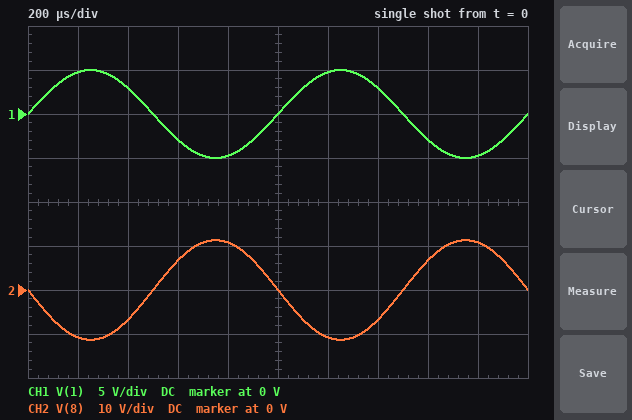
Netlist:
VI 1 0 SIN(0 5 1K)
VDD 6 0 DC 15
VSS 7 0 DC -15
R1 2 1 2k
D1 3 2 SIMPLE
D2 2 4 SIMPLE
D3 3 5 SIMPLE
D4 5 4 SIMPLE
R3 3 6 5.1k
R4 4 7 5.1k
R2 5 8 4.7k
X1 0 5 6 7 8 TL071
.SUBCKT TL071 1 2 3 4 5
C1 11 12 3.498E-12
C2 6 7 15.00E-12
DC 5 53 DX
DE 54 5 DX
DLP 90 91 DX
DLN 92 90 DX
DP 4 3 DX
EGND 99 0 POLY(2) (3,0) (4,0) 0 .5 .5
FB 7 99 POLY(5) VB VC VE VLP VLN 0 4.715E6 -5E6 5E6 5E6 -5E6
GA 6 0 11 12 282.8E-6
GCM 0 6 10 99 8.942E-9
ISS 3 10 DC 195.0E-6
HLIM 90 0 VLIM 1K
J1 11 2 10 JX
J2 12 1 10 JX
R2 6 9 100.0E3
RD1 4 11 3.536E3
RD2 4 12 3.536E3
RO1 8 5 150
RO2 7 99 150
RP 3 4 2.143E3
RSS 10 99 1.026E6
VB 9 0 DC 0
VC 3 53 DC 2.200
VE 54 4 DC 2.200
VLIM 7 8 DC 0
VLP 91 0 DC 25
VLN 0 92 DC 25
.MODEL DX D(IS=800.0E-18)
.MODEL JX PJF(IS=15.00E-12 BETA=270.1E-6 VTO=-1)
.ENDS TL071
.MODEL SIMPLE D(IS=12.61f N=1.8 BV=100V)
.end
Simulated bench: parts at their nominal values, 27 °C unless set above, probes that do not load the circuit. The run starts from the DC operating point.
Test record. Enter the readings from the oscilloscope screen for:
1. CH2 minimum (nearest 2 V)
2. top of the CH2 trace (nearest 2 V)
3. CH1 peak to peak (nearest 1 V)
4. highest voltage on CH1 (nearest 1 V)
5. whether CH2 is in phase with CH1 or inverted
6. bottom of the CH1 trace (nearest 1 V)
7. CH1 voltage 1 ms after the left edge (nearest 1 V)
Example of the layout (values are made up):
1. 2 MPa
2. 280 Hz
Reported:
1. -12 V
2. 12 V
3. 10 V
4. 5 V
5. inverted
6. -5 V
7. 0 V
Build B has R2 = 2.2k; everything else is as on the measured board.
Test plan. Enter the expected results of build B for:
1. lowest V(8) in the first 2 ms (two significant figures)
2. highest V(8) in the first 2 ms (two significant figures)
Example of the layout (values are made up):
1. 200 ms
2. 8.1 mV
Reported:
1. -5.3 V
2. 5.3 V
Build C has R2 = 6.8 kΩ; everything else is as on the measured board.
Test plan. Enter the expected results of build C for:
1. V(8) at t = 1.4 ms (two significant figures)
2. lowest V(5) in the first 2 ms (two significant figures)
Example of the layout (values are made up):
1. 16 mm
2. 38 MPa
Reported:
1. -9.8 V
2. -430 mV
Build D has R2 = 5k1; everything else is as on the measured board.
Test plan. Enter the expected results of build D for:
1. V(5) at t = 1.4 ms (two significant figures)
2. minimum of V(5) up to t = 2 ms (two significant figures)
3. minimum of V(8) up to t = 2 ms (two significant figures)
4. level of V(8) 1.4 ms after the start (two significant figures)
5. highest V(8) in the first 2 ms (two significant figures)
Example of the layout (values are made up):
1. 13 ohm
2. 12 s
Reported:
1. -2.9 mV
2. -3.7 mV
3. -12 V
4. -7.3 V
5. 12 V
